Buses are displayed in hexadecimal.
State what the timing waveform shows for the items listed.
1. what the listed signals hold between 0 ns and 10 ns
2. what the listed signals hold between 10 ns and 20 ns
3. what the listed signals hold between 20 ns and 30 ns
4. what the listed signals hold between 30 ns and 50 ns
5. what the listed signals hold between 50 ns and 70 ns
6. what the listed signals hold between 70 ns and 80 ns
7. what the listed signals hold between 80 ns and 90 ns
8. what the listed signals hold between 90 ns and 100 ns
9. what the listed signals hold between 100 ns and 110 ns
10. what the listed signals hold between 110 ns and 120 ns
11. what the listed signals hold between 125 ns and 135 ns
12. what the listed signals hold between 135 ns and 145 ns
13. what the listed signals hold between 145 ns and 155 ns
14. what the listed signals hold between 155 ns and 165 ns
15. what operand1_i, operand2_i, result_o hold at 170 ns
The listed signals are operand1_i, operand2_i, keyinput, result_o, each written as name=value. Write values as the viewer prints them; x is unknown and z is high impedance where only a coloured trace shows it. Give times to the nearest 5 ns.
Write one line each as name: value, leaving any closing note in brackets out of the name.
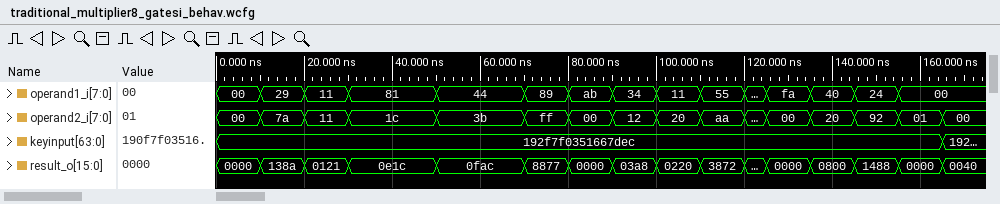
what the listed signals hold between 0 ns and 10 ns: operand1_i=00, operand2_i=00, keyinput=192f7f0351667dec, result_o=0000
what the listed signals hold between 10 ns and 20 ns: operand1_i=29, operand2_i=7a, keyinput=192f7f0351667dec, result_o=138a
what the listed signals hold between 20 ns and 30 ns: operand1_i=11, operand2_i=11, keyinput=192f7f0351667dec, result_o=0121
what the listed signals hold between 30 ns and 50 ns: operand1_i=81, operand2_i=1c, keyinput=192f7f0351667dec, result_o=0e1c
what the listed signals hold between 50 ns and 70 ns: operand1_i=44, operand2_i=3b, keyinput=192f7f0351667dec, result_o=0fac
what the listed signals hold between 70 ns and 80 ns: operand1_i=89, operand2_i=ff, keyinput=192f7f0351667dec, result_o=8877
what the listed signals hold between 80 ns and 90 ns: operand1_i=ab, operand2_i=00, keyinput=192f7f0351667dec, result_o=0000
what the listed signals hold between 90 ns and 100 ns: operand1_i=34, operand2_i=12, keyinput=192f7f0351667dec, result_o=03a8
what the listed signals hold between 100 ns and 110 ns: operand1_i=11, operand2_i=20, keyinput=192f7f0351667dec, result_o=0220
what the listed signals hold between 110 ns and 120 ns: operand1_i=55, operand2_i=aa, keyinput=192f7f0351667dec, result_o=3872
what the listed signals hold between 125 ns and 135 ns: operand1_i=fa, operand2_i=00, keyinput=192f7f0351667dec, result_o=0000
what the listed signals hold between 135 ns and 145 ns: operand1_i=40, operand2_i=20, keyinput=192f7f0351667dec, result_o=0800
what the listed signals hold between 145 ns and 155 ns: operand1_i=24, operand2_i=92, keyinput=192f7f0351667dec, result_o=1488
what the listed signals hold between 155 ns and 165 ns: operand1_i=00, operand2_i=01, keyinput=192f7f0351667dec, result_o=0000
what operand1_i, operand2_i, result_o hold at 170 ns: operand1_i=00, operand2_i=00, result_o=0040
